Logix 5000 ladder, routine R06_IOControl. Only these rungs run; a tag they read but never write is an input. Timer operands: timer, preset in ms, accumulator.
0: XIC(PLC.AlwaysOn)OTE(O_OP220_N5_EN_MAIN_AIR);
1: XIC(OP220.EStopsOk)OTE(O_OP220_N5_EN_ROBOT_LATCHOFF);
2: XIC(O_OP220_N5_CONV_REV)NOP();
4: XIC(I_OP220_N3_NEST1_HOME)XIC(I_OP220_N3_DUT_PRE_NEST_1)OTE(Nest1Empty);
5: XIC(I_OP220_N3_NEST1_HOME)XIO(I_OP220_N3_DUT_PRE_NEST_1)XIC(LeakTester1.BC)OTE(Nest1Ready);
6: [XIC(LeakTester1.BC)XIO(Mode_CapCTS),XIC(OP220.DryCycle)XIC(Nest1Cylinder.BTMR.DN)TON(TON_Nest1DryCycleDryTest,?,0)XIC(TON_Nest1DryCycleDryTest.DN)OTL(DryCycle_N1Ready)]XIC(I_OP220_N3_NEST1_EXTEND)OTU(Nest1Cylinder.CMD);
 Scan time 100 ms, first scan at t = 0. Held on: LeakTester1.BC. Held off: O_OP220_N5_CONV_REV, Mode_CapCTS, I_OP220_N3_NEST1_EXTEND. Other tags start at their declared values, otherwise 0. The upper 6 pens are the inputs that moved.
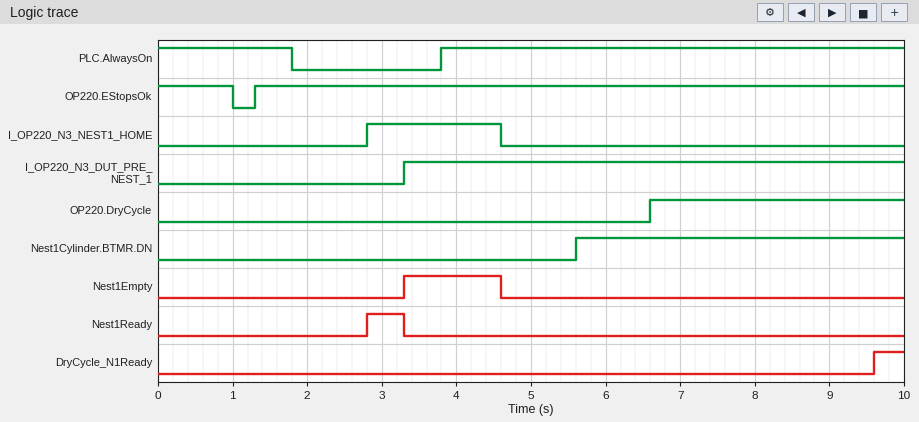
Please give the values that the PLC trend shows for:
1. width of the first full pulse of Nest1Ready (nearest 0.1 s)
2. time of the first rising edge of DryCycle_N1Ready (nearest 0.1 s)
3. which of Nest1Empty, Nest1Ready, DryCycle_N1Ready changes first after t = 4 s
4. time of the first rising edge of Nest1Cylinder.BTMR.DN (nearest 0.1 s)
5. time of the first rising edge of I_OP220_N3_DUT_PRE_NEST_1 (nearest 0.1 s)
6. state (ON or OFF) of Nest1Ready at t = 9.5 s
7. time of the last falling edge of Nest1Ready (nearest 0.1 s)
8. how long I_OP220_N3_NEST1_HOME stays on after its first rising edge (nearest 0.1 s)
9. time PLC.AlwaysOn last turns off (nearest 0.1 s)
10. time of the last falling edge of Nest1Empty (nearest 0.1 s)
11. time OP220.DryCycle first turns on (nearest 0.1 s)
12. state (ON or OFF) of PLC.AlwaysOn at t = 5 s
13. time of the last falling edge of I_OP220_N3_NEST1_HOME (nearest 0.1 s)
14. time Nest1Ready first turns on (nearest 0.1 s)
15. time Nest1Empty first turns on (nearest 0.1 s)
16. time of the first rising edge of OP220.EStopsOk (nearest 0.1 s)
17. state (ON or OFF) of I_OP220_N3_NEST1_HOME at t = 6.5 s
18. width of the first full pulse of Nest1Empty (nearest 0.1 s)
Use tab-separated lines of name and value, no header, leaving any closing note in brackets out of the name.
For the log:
width of the first full pulse of Nest1Ready	0.5 s
time of the first rising edge of DryCycle_N1Ready	9.6 s
which of Nest1Empty, Nest1Ready, DryCycle_N1Ready changes first after t = 4 s	Nest1Empty
time of the first rising edge of Nest1Cylinder.BTMR.DN	5.6 s
time of the first rising edge of I_OP220_N3_DUT_PRE_NEST_1	3.3 s
state (ON or OFF) of Nest1Ready at t = 9.5 s	OFF
time of the last falling edge of Nest1Ready	3.3 s
how long I_OP220_N3_NEST1_HOME stays on after its first rising edge	1.8 s
time PLC.AlwaysOn last turns off	1.8 s
time of the last falling edge of Nest1Empty	4.6 s
time OP220.DryCycle first turns on	6.6 s
state (ON or OFF) of PLC.AlwaysOn at t = 5 s	ON
time of the last falling edge of I_OP220_N3_NEST1_HOME	4.6 s
time Nest1Ready first turns on	2.8 s
time Nest1Empty first turns on	3.3 s
time of the first rising edge of OP220.EStopsOk	1.3 s
state (ON or OFF) of I_OP220_N3_NEST1_HOME at t = 6.5 s	OFF
width of the first full pulse of Nest1Empty	1.3 s
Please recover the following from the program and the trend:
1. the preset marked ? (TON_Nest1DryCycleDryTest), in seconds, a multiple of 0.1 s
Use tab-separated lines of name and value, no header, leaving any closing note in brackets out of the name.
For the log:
the preset marked ? (TON_Nest1DryCycleDryTest), in seconds, a multiple of 0.1 s	3.0 s
